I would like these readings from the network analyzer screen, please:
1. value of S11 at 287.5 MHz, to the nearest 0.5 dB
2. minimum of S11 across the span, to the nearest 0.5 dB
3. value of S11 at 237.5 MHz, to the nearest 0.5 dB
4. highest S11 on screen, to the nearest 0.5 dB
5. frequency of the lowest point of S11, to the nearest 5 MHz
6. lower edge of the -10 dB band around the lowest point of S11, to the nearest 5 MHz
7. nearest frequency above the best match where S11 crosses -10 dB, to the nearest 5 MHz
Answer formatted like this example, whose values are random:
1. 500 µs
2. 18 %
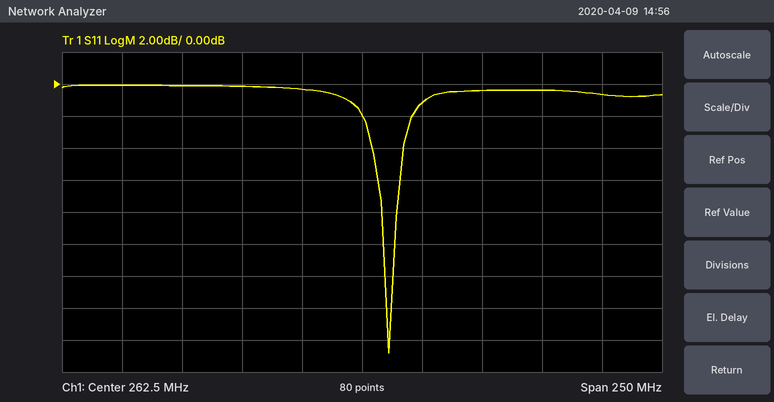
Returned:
1. -1.0 dB
2. -17.0 dB
3. -0.5 dB
4. 0.0 dB
5. 275 MHz
6. 270 MHz
7. 275 MHz
